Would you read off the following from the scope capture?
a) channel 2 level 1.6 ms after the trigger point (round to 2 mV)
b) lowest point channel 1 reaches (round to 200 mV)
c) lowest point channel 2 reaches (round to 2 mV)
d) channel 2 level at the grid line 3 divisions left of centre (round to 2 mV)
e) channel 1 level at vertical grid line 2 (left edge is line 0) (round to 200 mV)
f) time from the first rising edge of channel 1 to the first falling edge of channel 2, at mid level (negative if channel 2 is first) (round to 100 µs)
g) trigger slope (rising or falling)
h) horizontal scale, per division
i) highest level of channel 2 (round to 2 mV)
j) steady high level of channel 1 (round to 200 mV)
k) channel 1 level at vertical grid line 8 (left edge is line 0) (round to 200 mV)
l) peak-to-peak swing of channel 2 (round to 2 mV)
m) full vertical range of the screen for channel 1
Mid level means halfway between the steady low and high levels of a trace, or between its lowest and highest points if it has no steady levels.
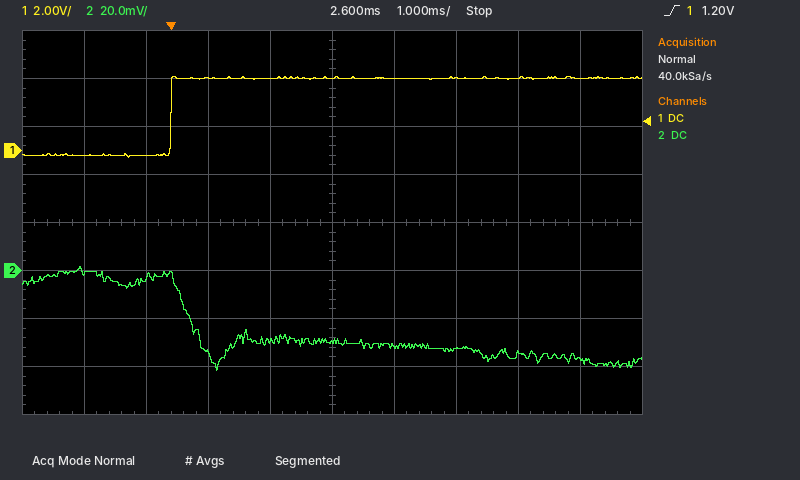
-30 mV
-200 mV
-42 mV
-2 mV
-200 mV
+300 µs
rising
1 ms
2 mV
3.0 V
3.0 V
44 mV
16 V
